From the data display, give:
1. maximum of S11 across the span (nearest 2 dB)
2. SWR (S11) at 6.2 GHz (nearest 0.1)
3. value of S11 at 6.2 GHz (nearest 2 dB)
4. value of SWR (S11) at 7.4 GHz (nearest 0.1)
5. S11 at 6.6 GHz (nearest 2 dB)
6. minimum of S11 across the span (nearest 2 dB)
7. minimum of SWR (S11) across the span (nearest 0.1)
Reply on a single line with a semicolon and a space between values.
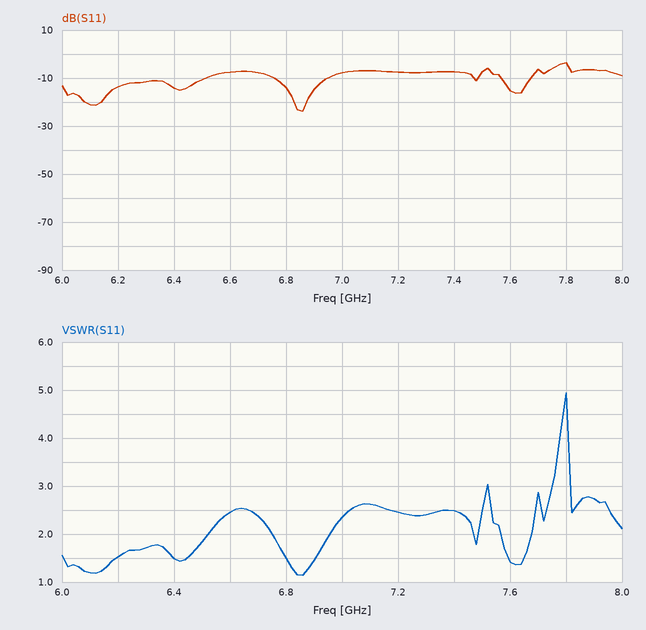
-4 dB; 1.5; -14 dB; 2.5; -8 dB; -24 dB; 1.1
